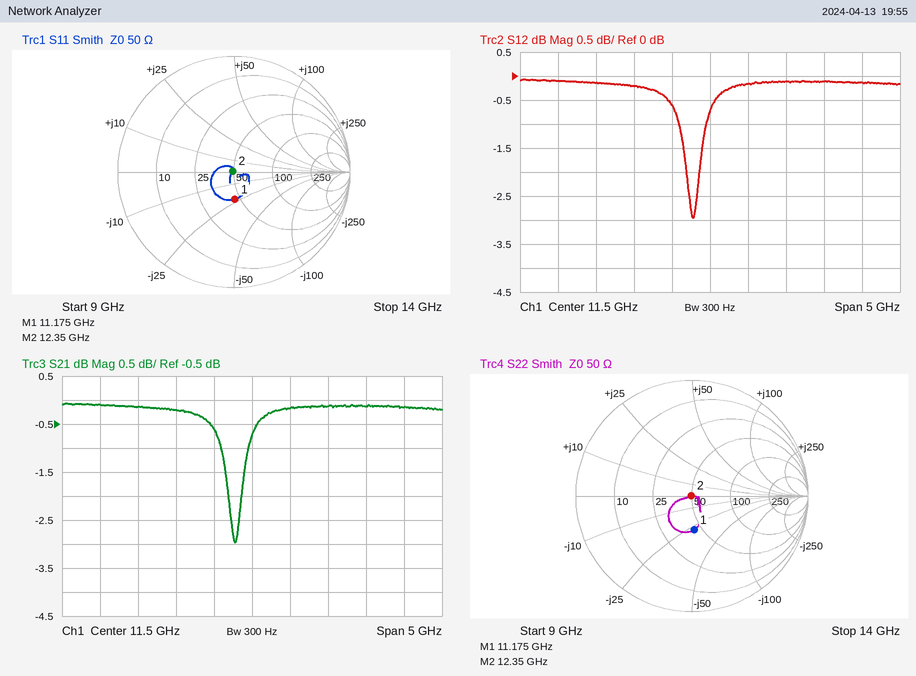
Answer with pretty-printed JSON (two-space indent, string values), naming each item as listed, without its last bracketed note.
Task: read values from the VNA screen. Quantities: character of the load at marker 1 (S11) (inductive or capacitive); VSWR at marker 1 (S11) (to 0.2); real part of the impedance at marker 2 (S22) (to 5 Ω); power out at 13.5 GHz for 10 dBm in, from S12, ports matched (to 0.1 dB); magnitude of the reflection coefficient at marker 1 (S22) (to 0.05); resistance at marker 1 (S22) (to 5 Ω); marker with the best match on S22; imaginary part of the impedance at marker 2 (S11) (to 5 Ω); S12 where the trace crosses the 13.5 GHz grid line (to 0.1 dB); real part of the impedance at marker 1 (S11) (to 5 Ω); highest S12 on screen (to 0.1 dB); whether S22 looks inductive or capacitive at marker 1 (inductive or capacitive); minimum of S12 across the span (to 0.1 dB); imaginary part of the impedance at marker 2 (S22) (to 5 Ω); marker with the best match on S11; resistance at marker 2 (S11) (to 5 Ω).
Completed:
{
  "character of the load at marker 1 (S11)": "capacitive",
  "VSWR at marker 1 (S11)": "1.6",
  "real part of the impedance at marker 2 (S22)": "50 Ω",
  "power out at 13.5 GHz for 10 dBm in, from S12, ports matched": "9.9 dBm",
  "magnitude of the reflection coefficient at marker 1 (S22)": "0.30",
  "resistance at marker 1 (S22)": "45 Ω",
  "marker with the best match on S22": "marker 2",
  "imaginary part of the impedance at marker 2 (S11)": "0 Ω",
  "S12 where the trace crosses the 13.5 GHz grid line": "-0.1 dB",
  "real part of the impedance at marker 1 (S11)": "45 Ω",
  "highest S12 on screen": "-0.1 dB",
  "whether S22 looks inductive or capacitive at marker 1": "capacitive",
  "minimum of S12 across the span": "-3.0 dB",
  "imaginary part of the impedance at marker 2 (S22)": "0 Ω",
  "marker with the best match on S11": "marker 2",
  "resistance at marker 2 (S11)": "50 Ω"
}
